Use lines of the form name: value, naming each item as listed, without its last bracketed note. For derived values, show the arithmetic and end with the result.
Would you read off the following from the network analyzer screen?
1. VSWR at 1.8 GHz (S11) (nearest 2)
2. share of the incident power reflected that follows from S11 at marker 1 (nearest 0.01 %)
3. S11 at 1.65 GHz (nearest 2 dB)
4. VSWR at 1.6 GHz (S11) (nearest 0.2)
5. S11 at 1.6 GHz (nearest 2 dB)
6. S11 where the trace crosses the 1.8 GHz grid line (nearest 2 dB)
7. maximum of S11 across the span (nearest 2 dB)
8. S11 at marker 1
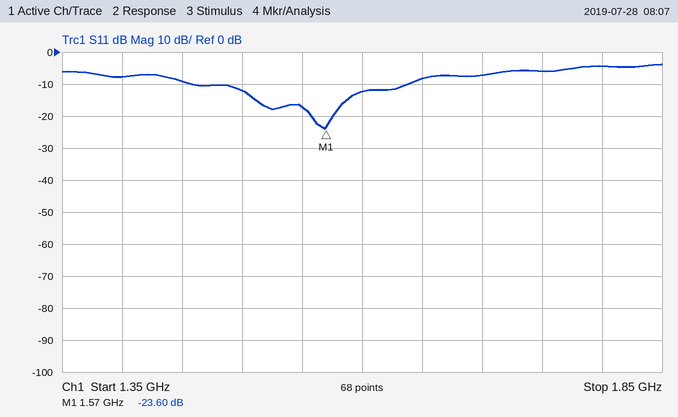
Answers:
VSWR at 1.8 GHz (S11): |Γ| = 10^(-4/20) = 0.6310; VSWR = (1 + 0.6310)/(1 − 0.6310) ≈ 4
share of the incident power reflected that follows from S11 at marker 1: 10^(-23.6/10) ≈ 0.44 %
S11 at 1.65 GHz: -8 dB
VSWR at 1.6 GHz (S11): |Γ| = 10^(-12/20) = 0.2512; VSWR = (1 + 0.2512)/(1 − 0.2512) ≈ 1.67, so 1.6 to the nearest 0.2
S11 at 1.6 GHz: -12 dB
S11 where the trace crosses the 1.8 GHz grid line: -4 dB
maximum of S11 across the span: -4 dB
S11 at marker 1: -23.60 dB
